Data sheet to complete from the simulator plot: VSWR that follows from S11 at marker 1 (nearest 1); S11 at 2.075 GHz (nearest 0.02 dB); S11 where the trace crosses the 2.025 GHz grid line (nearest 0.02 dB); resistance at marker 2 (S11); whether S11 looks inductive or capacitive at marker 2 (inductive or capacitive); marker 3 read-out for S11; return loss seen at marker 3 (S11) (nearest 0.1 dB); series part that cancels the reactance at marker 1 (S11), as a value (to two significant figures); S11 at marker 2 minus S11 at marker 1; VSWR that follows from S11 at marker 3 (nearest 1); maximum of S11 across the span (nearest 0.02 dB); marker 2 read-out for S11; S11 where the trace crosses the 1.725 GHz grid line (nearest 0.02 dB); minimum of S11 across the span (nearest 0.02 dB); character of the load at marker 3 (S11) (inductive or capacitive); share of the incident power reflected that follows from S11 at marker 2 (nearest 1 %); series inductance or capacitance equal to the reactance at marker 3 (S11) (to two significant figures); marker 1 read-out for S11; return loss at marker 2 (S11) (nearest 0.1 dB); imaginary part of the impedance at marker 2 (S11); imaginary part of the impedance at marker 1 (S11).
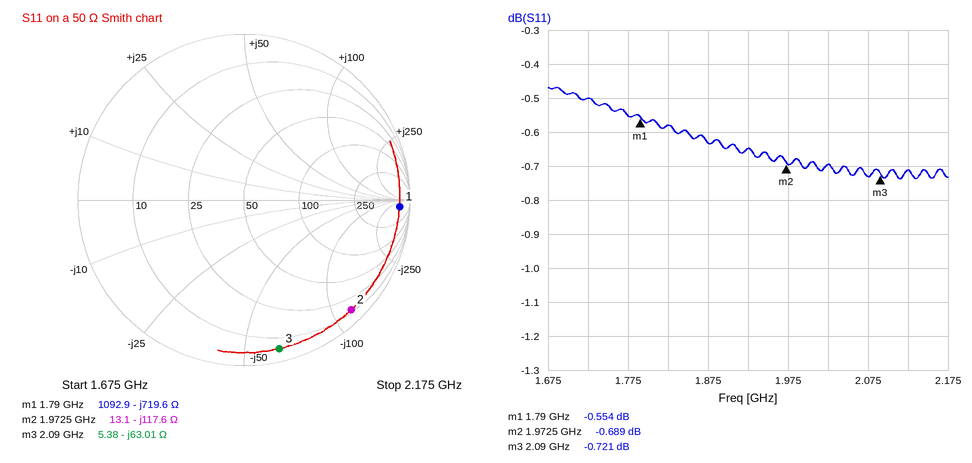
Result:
31
-0.74 dB
-0.70 dB
13.1 Ω
capacitive
-0.721 dB
0.7 dB
64 nH
-0.135 dB
24
-0.46 dB
-0.689 dB
-0.50 dB
-0.74 dB
capacitive
85 %
1.2 pF
-0.554 dB
0.7 dB
-117.6 Ω
-719.6 Ω
